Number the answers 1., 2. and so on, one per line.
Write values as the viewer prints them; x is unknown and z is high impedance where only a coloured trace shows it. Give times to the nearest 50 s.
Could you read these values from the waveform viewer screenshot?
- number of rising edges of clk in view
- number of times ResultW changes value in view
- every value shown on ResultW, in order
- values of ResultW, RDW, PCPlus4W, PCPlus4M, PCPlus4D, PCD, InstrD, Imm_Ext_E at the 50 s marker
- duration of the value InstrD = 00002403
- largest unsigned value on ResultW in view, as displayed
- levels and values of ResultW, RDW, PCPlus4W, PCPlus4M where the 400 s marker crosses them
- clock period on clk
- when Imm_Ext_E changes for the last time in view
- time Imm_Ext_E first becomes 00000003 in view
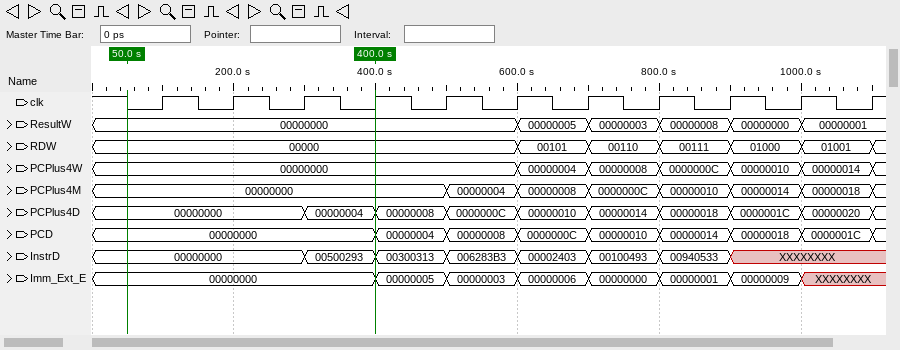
1. 11
2. 5
3. 00000000, 00000005, 00000003, 00000008, 00000000, 00000001
4. ResultW=00000000, RDW=00000, PCPlus4W=00000000, PCPlus4M=00000000, PCPlus4D=00000000, PCD=00000000, InstrD=00000000, Imm_Ext_E=00000000
5. 100 s
6. 00000008
7. ResultW=00000000, RDW=00000, PCPlus4W=00000000, PCPlus4M=00000000
8. 100 s
9. 1000 s
10. 500 s
